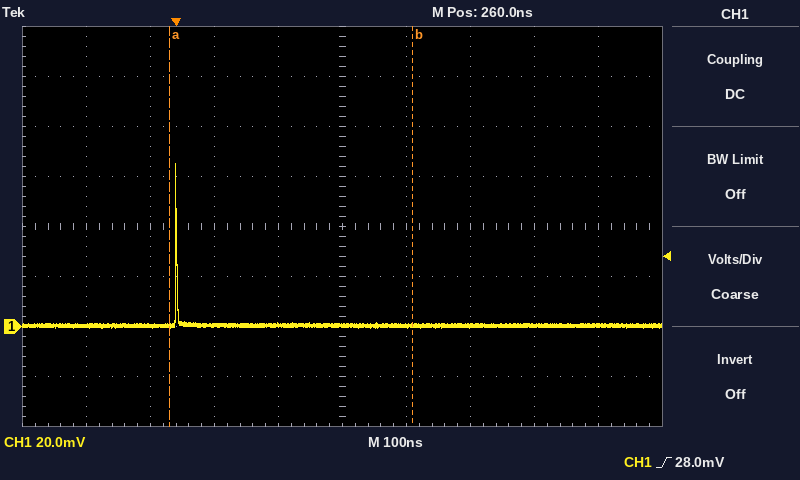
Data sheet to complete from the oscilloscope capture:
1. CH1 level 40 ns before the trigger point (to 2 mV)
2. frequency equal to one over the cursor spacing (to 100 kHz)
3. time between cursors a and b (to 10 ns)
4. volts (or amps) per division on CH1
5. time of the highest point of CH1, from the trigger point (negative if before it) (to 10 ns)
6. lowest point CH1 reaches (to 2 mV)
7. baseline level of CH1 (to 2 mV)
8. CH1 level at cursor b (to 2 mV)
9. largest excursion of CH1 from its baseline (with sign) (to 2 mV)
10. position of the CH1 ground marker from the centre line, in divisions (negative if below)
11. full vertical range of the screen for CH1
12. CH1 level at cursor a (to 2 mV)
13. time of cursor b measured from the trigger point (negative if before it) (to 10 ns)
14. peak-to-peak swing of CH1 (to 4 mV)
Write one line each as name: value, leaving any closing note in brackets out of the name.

CH1 level 40 ns before the trigger point: 0 mV
frequency equal to one over the cursor spacing: 2.6 MHz
time between cursors a and b: 380 ns
volts (or amps) per division on CH1: 20 mV
time of the highest point of CH1, from the trigger point (negative if before it): 0 ns
lowest point CH1 reaches: 0 mV
baseline level of CH1: 0 mV
CH1 level at cursor b: 0 mV
largest excursion of CH1 from its baseline (with sign): +64 mV
position of the CH1 ground marker from the centre line, in divisions: -2.0 div
full vertical range of the screen for CH1: 160 mV
CH1 level at cursor a: 0 mV
time of cursor b measured from the trigger point (negative if before it): +370 ns
peak-to-peak swing of CH1: 64 mV
